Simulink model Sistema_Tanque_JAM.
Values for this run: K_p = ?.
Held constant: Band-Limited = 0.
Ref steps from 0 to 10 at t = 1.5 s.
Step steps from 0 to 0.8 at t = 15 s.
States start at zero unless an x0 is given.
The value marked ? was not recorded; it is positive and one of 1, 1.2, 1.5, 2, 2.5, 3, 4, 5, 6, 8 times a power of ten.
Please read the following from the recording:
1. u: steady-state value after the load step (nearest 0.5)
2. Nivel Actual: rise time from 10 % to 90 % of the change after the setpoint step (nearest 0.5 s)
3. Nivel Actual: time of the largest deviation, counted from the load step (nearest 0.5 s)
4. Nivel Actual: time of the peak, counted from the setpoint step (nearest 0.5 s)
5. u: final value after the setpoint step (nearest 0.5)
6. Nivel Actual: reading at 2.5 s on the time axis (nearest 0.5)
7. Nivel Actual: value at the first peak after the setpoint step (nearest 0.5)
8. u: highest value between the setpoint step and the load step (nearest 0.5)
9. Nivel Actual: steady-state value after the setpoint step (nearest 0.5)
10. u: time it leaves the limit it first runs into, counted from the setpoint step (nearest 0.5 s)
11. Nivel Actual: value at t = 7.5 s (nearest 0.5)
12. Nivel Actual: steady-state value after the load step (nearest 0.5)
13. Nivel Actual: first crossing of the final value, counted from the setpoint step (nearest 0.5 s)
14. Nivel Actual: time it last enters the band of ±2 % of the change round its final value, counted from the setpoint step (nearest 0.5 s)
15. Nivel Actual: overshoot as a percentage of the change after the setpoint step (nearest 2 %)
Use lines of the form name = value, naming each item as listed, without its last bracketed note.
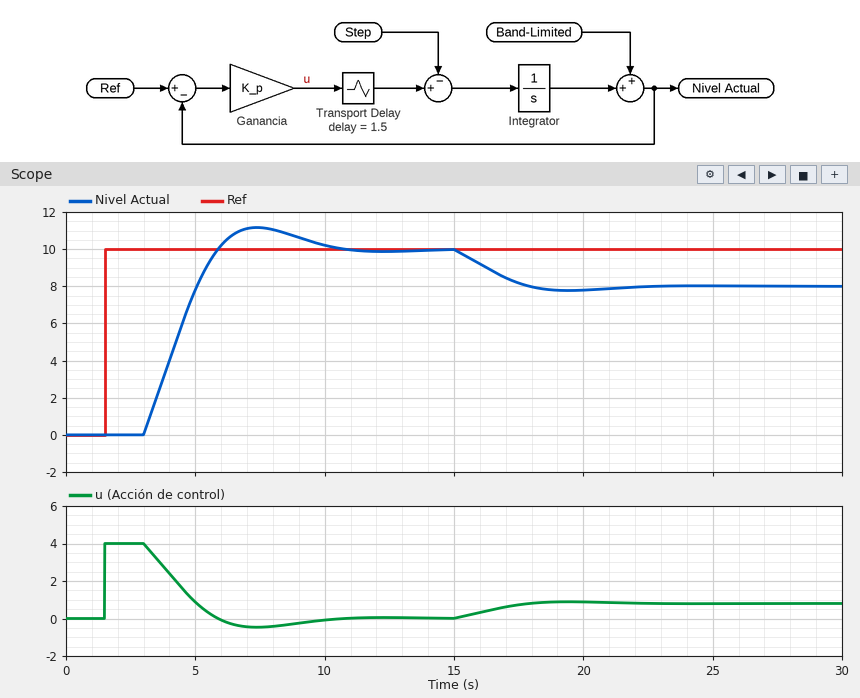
u: steady-state value after the load step = 1.0
Nivel Actual: rise time from 10 % to 90 % of the change after the setpoint step = 2.0 s
Nivel Actual: time of the largest deviation, counted from the load step = 4.5 s
Nivel Actual: time of the peak, counted from the setpoint step = 6.0 s
u: final value after the setpoint step = 0.0
Nivel Actual: reading at 2.5 s on the time axis = 0.0
Nivel Actual: value at the first peak after the setpoint step = 11.0
u: highest value between the setpoint step and the load step = 4.0
Nivel Actual: steady-state value after the setpoint step = 10.0
u: time it leaves the limit it first runs into, counted from the setpoint step = 1.5 s
Nivel Actual: value at t = 7.5 s = 11.0
Nivel Actual: steady-state value after the load step = 8.0
Nivel Actual: first crossing of the final value, counted from the setpoint step = 4.5 s
Nivel Actual: time it last enters the band of ±2 % of the change round its final value, counted from the setpoint step = 8.5 s
Nivel Actual: overshoot as a percentage of the change after the setpoint step = 12 %
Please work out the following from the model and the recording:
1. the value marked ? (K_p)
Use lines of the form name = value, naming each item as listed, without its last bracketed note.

the value marked ? = 0.4
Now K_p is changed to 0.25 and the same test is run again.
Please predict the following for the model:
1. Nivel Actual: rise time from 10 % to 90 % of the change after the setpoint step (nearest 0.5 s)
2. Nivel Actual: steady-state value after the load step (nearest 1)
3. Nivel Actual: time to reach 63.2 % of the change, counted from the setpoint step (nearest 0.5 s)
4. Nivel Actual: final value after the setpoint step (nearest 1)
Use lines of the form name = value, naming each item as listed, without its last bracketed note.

Nivel Actual: rise time from 10 % to 90 % of the change after the setpoint step = 5.0 s
Nivel Actual: steady-state value after the load step = 7
Nivel Actual: time to reach 63.2 % of the change, counted from the setpoint step = 4.0 s
Nivel Actual: final value after the setpoint step = 10
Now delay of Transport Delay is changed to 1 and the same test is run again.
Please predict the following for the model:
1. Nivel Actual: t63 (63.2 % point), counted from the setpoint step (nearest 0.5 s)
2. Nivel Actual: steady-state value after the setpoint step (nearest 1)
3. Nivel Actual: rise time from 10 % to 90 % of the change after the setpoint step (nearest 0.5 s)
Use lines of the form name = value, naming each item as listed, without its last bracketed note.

Nivel Actual: t63 (63.2 % point), counted from the setpoint step = 2.5 s
Nivel Actual: steady-state value after the setpoint step = 10
Nivel Actual: rise time from 10 % to 90 % of the change after the setpoint step = 3.0 s
